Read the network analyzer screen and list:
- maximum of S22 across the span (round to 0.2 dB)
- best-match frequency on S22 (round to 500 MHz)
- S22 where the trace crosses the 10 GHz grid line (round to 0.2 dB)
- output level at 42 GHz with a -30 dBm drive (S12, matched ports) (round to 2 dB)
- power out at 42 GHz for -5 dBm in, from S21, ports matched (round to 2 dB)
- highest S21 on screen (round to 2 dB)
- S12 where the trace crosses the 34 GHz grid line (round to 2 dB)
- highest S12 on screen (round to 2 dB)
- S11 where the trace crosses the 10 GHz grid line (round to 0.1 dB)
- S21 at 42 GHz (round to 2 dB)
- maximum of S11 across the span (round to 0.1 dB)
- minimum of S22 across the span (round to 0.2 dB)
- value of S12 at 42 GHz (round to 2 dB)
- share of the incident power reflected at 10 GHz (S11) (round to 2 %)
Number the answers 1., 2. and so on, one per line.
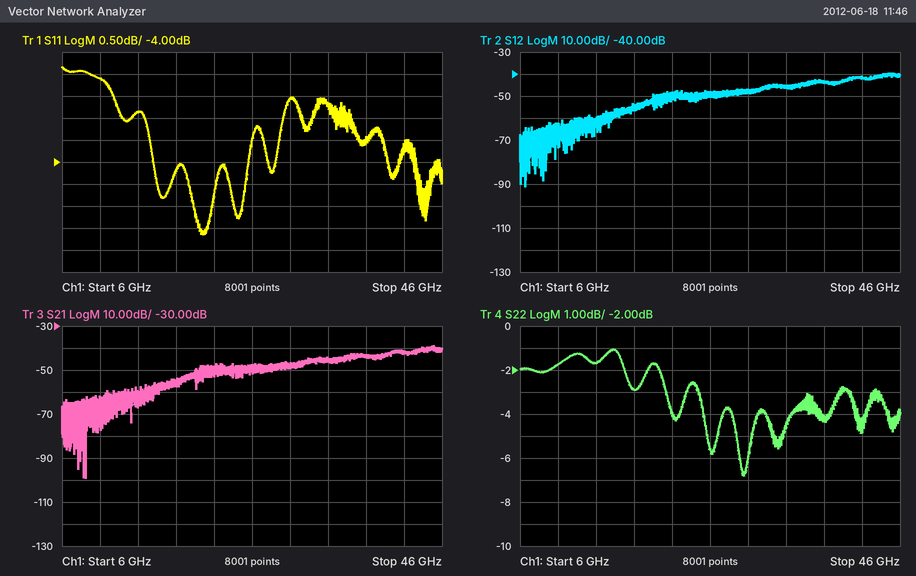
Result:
1. -1.0 dB
2. 29.5 GHz
3. -1.8 dB
4. -72 dBm
5. -46 dBm
6. -38 dB
7. -46 dB
8. -40 dB
9. -2.1 dB
10. -42 dB
11. -1.8 dB
12. -6.8 dB
13. -42 dB
14. 62 %
